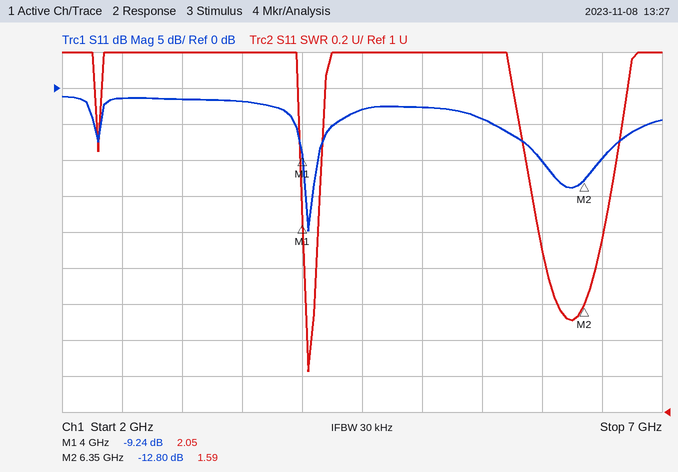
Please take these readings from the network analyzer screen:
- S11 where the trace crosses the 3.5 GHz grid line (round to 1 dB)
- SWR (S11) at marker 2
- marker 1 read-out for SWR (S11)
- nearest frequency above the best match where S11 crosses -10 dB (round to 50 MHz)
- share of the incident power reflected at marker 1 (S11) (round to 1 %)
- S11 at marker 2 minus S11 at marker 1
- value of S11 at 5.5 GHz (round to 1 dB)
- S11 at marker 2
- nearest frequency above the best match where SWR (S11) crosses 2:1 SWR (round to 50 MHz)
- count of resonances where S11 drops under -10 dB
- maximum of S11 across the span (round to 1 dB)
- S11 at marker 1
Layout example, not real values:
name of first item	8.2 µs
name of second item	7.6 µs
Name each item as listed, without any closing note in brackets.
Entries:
S11 where the trace crosses the 3.5 GHz grid line	-2 dB
SWR (S11) at marker 2	1.59
marker 1 read-out for SWR	2.05
nearest frequency above the best match where S11 crosses -10 dB	4.15 GHz
share of the incident power reflected at marker 1 (S11)	12 %
S11 at marker 2 minus S11 at marker 1	-3.56 dB
value of S11 at 5.5 GHz	-4 dB
S11 at marker 2	-12.80 dB
nearest frequency above the best match where SWR (S11) crosses 2:1 SWR	4.15 GHz
count of resonances where S11 drops under -10 dB	2
maximum of S11 across the span	-1 dB
S11 at marker 1	-9.24 dB
